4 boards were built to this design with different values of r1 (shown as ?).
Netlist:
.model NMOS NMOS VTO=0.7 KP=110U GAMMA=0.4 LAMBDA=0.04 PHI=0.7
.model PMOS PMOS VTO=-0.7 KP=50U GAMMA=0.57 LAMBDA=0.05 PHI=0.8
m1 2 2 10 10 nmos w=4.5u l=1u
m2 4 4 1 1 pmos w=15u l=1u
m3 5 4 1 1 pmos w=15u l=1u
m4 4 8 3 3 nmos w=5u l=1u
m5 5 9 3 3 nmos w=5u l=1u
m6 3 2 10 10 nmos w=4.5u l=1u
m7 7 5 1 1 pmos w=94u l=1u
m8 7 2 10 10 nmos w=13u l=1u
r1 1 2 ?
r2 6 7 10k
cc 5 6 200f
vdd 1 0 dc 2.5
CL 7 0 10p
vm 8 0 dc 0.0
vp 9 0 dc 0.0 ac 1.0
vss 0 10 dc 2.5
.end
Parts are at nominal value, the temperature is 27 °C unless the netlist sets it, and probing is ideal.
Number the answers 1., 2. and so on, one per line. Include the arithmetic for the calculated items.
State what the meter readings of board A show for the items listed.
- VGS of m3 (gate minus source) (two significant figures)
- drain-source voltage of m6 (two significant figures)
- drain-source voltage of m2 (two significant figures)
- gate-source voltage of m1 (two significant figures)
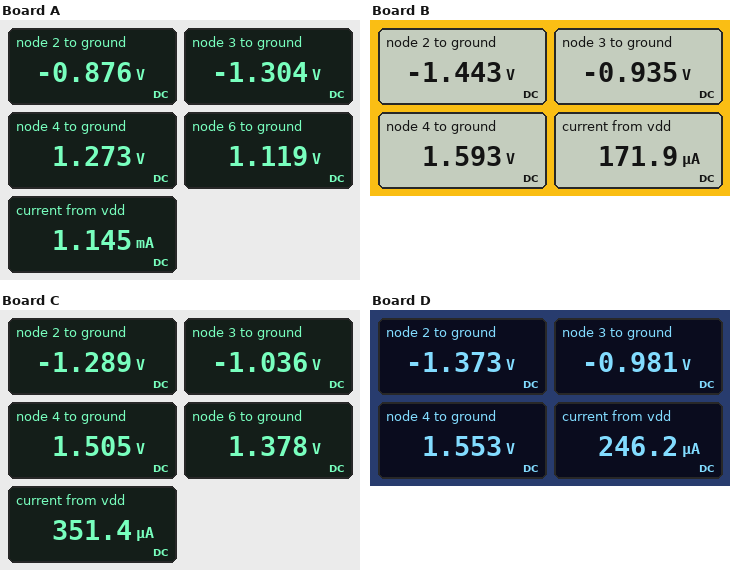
1. 1.273 V - 2.5 V = -1.2 V
2. -1.304 V - (-2.5 V) = 1.2 V
3. 1.273 V - 2.5 V = -1.2 V
4. -876 mV - (-2.5 V) = 1.6 V
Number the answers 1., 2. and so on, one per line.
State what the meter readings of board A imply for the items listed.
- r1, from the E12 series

1. 15 kΩ
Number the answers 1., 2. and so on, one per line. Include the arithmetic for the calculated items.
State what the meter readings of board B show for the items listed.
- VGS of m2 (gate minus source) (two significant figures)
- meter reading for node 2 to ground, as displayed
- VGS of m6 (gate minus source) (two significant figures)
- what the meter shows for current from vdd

1. 1.593 V - 2.5 V = -910 mV
2. -1.443 V
3. -1.443 V - (-2.5 V) = 1.1 V
4. 171.9 µA
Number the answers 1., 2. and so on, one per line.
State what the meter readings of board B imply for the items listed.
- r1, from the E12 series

1. 120 kΩ
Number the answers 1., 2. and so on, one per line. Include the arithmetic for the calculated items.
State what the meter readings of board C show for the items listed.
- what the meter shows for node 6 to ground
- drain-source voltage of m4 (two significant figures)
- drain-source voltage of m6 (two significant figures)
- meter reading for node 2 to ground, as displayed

1. 1.378 V
2. 1.505 V - (-1.036 V) = 2.5 V
3. -1.036 V - (-2.5 V) = 1.5 V
4. -1.289 V
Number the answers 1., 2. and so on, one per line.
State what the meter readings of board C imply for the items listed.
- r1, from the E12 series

1. 56 kΩ
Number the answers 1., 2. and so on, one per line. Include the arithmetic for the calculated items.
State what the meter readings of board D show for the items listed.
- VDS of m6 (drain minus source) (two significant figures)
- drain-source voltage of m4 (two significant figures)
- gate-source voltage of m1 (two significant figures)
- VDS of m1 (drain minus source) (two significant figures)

1. -981 mV - (-2.5 V) = 1.5 V
2. 1.553 V - (-981 mV) = 2.5 V
3. -1.373 V - (-2.5 V) = 1.1 V
4. -1.373 V - (-2.5 V) = 1.1 V
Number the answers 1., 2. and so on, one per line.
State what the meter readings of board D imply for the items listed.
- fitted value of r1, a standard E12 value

1. 82 kΩ
